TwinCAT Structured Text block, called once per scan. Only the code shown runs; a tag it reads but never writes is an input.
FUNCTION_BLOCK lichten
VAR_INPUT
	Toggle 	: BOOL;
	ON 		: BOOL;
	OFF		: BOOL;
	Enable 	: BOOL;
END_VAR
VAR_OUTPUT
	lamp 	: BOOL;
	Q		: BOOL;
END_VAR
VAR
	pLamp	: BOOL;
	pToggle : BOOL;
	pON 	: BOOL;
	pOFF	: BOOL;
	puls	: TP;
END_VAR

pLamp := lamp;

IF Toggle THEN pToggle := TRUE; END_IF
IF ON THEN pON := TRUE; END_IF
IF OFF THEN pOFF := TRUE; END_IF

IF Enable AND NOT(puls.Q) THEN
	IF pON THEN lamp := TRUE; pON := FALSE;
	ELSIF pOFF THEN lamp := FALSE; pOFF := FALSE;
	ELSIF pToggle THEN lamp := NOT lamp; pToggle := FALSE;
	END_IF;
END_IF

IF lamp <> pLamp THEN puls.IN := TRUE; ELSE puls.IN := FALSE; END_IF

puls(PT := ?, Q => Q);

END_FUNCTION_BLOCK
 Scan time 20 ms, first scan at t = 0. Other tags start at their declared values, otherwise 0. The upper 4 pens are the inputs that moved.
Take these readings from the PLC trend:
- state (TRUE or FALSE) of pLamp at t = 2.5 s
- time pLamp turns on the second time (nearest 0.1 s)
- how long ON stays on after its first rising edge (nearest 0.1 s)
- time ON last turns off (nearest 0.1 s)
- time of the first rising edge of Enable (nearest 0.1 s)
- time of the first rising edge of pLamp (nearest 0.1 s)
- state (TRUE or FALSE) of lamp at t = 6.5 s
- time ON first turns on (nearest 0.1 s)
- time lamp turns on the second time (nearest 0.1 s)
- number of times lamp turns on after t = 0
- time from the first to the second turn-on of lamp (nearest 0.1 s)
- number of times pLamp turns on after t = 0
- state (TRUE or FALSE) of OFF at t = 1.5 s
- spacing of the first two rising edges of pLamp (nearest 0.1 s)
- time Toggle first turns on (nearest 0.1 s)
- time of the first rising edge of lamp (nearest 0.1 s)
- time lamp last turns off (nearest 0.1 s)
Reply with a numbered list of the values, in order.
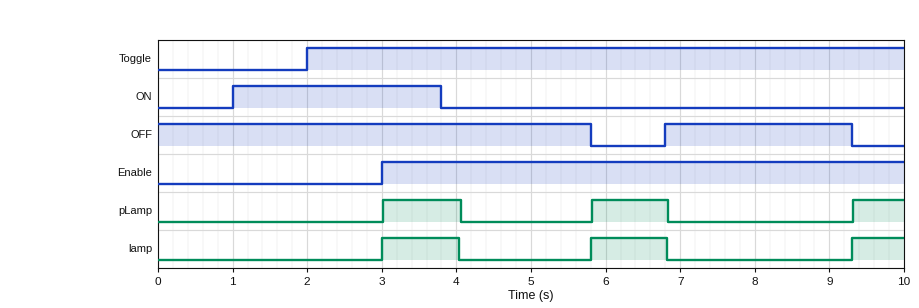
1. FALSE
2. 5.8 s
3. 2.8 s
4. 3.8 s
5. 3.0 s
6. 3.0 s
7. TRUE
8. 1.0 s
9. 5.8 s
10. 3
11. 2.8 s
12. 3
13. TRUE
14. 2.8 s
15. 2.0 s
16. 3.0 s
17. 6.8 s
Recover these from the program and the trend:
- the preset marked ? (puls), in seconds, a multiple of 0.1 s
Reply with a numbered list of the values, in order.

1. 1.0 s
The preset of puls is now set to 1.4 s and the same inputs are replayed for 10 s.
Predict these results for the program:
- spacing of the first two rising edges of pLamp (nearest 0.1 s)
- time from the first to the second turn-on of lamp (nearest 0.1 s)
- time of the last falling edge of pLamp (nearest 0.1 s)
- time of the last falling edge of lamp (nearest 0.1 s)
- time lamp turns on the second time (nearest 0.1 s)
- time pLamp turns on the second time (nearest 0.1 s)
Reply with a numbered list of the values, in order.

1. 2.9 s
2. 2.9 s
3. 7.3 s
4. 7.3 s
5. 5.9 s
6. 5.9 s
